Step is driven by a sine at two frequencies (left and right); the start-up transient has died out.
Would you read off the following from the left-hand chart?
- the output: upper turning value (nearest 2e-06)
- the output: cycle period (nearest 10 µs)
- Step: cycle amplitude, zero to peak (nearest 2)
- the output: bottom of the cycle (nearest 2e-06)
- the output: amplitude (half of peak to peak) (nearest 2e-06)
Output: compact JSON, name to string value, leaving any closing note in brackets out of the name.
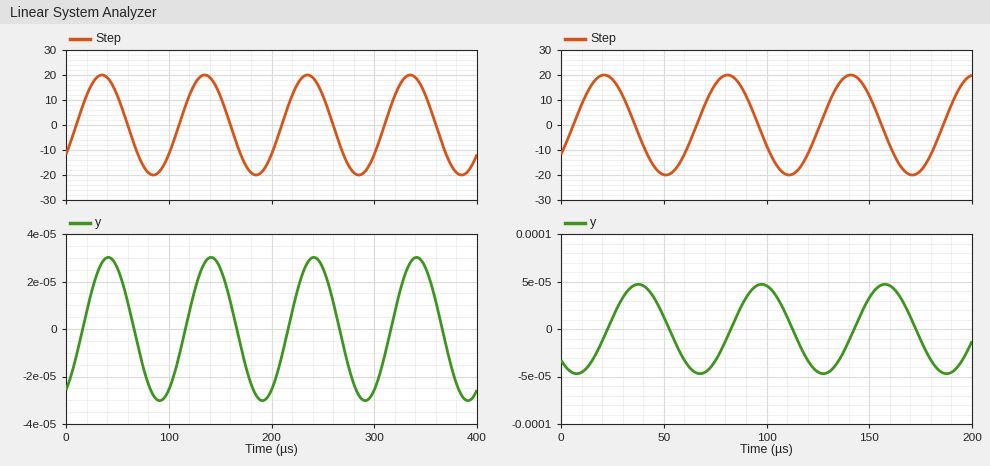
{"the output: upper turning value": "0.000030", "the output: cycle period": "100 µs", "Step: cycle amplitude, zero to peak": "20", "the output: bottom of the cycle": "-0.000030", "the output: amplitude (half of peak to peak)": "0.000030"}
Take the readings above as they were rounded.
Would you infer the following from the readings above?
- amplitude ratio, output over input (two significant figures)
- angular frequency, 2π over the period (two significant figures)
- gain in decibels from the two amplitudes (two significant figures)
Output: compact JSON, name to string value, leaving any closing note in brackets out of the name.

{"amplitude ratio, output over input": "0.0000015", "angular frequency, 2π over the period": "0.063 rad/µs", "gain in decibels from the two amplitudes": "-120 dB"}
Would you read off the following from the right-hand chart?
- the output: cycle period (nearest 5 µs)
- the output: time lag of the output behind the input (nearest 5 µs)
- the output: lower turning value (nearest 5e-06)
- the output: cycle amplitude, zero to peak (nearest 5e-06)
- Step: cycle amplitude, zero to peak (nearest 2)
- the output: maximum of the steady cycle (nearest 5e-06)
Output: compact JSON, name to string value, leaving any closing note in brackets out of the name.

{"the output: cycle period": "60 µs", "the output: time lag of the output behind the input": "15 µs", "the output: lower turning value": "-0.000045", "the output: cycle amplitude, zero to peak": "0.000045", "Step: cycle amplitude, zero to peak": "20", "the output: maximum of the steady cycle": "0.000045"}
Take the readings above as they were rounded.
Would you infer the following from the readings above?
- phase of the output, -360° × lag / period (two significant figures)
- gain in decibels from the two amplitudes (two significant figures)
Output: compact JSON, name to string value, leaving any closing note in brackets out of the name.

{"phase of the output, -360° × lag / period": "-90°", "gain in decibels from the two amplitudes": "-110 dB"}
